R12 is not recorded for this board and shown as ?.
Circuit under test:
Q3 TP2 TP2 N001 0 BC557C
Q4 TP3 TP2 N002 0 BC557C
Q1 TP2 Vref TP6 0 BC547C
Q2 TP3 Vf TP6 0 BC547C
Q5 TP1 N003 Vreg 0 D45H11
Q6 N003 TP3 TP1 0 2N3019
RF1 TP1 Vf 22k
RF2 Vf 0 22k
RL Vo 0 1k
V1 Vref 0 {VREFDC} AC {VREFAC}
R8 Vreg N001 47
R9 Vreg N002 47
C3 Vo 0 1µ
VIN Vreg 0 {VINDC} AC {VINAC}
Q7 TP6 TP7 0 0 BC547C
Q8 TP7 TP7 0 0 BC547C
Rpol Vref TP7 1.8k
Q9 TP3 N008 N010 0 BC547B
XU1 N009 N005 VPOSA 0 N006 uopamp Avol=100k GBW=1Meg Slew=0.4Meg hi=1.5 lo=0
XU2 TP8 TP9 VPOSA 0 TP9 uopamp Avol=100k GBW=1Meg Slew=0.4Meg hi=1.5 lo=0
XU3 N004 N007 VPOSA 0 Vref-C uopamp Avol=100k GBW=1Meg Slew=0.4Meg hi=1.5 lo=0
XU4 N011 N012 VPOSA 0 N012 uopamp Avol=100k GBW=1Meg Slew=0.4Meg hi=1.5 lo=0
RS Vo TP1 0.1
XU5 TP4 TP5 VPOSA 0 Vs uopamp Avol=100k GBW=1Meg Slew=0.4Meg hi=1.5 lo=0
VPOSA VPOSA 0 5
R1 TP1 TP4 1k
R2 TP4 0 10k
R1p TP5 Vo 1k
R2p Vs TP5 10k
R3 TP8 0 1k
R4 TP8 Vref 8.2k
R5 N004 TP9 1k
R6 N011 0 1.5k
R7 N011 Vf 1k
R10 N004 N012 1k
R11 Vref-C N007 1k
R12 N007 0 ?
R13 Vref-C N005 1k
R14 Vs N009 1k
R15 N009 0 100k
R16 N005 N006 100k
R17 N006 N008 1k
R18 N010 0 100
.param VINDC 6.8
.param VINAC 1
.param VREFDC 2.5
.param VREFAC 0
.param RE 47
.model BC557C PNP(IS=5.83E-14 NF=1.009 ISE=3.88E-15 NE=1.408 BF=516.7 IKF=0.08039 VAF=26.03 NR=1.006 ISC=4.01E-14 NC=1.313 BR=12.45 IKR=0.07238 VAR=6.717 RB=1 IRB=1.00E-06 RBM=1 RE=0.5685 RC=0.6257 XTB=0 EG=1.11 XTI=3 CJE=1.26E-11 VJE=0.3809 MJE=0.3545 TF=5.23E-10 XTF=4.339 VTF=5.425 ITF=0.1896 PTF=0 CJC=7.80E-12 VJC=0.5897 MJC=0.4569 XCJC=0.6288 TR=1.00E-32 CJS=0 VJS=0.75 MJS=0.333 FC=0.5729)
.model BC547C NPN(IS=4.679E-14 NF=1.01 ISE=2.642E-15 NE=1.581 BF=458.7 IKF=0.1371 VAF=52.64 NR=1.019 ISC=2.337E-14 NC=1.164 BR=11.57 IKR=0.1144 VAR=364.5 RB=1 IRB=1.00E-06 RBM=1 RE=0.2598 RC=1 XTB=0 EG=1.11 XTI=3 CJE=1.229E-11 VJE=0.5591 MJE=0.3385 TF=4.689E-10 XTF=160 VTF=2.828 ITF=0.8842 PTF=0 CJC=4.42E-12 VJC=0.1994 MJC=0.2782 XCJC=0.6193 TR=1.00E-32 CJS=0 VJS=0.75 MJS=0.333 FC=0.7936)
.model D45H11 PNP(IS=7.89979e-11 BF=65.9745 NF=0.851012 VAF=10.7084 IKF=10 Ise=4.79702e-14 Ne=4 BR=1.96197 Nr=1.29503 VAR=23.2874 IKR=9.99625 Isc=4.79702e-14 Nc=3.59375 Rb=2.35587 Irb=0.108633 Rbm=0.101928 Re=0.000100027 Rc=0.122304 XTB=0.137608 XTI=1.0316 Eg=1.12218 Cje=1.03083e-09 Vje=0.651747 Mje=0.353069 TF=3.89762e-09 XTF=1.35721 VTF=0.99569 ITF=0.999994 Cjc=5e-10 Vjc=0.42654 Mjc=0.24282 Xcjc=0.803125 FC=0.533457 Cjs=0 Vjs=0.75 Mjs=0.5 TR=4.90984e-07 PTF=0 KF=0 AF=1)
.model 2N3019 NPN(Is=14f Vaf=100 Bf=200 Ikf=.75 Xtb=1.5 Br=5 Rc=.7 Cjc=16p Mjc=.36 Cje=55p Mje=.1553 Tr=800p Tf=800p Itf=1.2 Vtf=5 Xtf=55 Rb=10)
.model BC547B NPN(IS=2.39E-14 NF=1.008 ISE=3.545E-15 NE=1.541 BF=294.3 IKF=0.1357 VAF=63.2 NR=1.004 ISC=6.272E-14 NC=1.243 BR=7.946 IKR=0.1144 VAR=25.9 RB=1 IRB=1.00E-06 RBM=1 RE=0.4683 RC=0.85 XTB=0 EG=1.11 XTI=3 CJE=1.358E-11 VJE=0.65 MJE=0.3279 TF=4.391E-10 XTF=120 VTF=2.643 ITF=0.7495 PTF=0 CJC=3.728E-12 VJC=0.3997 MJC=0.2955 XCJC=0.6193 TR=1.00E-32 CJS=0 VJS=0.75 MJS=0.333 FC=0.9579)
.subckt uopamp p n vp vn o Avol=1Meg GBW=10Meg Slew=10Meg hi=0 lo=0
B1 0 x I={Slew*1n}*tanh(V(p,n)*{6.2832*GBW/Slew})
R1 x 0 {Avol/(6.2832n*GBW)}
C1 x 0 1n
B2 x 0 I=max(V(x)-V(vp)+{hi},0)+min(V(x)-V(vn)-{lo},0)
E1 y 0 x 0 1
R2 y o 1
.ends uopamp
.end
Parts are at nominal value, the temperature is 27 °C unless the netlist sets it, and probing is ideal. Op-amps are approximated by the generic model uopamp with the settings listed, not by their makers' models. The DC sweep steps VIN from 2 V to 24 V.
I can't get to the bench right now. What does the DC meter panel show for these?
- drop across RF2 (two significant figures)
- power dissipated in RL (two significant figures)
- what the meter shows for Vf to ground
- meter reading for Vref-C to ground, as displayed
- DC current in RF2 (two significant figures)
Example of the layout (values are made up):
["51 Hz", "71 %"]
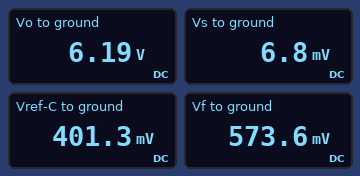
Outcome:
["570 mV", "38 mW", "573.6 mV", "401.3 mV", "26 µA"]
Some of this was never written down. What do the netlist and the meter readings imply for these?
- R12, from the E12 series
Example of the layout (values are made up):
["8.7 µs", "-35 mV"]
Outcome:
["3.3 kΩ"]
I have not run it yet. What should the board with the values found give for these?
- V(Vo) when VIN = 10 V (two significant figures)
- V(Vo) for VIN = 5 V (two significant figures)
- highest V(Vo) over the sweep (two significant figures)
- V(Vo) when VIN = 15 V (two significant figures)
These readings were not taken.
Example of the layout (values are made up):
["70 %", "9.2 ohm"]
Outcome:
["9.4 V", "4.4 V", "23 V", "14 V"]
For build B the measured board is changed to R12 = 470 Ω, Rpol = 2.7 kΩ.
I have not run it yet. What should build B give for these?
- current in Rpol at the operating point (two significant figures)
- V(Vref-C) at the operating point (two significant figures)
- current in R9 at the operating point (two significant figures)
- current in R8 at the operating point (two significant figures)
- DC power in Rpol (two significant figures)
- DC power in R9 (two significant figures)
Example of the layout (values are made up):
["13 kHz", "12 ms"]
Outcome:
["700 µA", "960 mV", "120 µA", "590 µA", "1.3 mW", "680 nW"]
